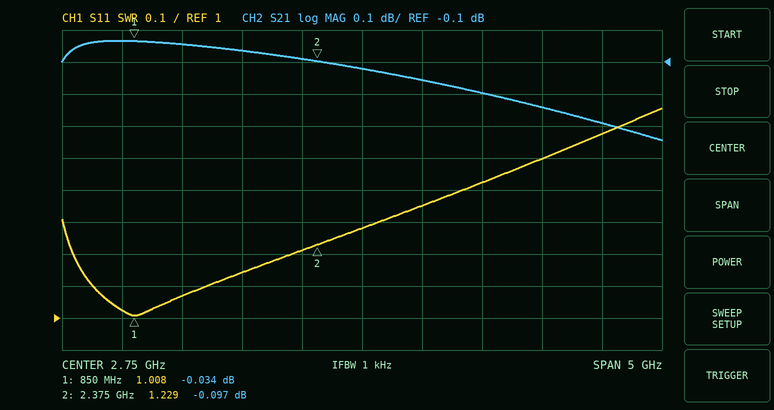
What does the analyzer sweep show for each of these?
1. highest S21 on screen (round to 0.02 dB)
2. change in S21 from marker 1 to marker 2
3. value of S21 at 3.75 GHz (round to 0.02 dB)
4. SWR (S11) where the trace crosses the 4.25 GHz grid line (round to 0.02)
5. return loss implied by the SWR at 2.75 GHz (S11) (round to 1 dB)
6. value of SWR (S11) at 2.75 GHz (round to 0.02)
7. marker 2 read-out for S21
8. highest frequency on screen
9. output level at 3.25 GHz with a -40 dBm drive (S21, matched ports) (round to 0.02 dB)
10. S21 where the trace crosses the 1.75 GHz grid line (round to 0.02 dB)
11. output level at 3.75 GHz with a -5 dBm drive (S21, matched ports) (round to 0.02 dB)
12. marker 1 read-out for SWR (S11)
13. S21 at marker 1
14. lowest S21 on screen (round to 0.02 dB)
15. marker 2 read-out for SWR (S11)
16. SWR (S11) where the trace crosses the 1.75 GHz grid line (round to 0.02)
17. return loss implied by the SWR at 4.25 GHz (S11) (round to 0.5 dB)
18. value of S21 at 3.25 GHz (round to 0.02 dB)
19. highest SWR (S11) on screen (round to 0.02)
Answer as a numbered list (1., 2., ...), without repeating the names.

1. -0.04 dB
2. -0.063 dB
3. -0.20 dB
4. 1.50
5. 18 dB
6. 1.28
7. -0.097 dB
8. 5.25 GHz
9. -40.16 dBm
10. -0.06 dB
11. -5.20 dBm
12. 1.008
13. -0.034 dB
14. -0.34 dB
15. 1.229
16. 1.14
17. 14.0 dB
18. -0.16 dB
19. 1.66
